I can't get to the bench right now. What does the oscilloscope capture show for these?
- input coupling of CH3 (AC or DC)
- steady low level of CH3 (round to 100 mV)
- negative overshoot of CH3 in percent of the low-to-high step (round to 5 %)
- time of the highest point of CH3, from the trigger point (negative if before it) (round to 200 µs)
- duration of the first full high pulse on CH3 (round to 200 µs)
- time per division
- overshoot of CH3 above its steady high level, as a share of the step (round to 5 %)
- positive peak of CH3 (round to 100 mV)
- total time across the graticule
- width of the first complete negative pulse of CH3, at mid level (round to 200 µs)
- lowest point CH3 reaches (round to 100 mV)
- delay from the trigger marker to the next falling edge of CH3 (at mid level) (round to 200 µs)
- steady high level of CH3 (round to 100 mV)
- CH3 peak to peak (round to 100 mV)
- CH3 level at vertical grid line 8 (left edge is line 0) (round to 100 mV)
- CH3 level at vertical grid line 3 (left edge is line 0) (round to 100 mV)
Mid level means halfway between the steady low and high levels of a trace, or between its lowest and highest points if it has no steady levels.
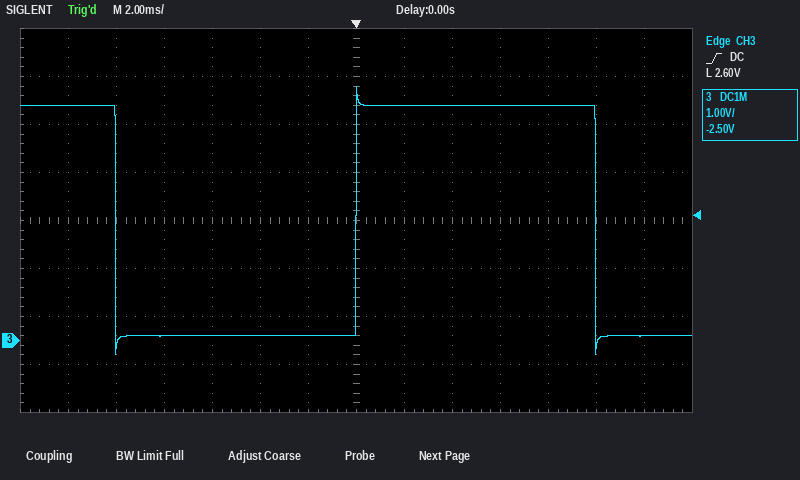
DC
100 mV
10 %
0.0 ms
10.0 ms
2 ms
10 %
5.3 V
28 ms
10.0 ms
-300 mV
10.0 ms
4.9 V
5.6 V
4.9 V
100 mV
